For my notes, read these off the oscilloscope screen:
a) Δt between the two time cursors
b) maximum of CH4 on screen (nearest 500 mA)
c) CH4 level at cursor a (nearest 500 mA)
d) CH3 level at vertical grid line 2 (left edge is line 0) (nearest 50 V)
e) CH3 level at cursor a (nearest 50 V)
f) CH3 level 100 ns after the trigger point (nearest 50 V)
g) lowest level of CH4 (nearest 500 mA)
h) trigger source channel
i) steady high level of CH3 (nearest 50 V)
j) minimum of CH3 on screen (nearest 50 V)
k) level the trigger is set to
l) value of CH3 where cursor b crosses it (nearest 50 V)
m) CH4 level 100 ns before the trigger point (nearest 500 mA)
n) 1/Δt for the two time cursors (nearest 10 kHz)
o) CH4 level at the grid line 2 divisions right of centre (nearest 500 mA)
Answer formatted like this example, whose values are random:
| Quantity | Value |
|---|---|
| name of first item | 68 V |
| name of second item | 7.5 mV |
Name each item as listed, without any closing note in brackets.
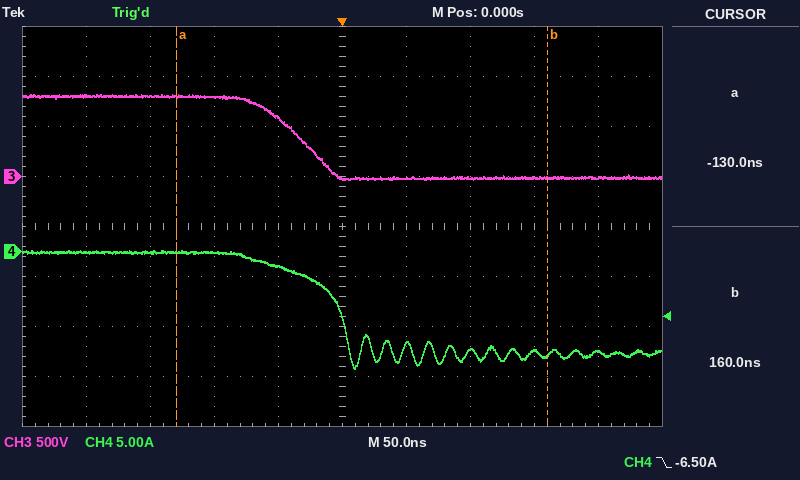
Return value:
| Quantity | Value |
|---|---|
| Δt between the two time cursors | 290 ns |
| maximum of CH4 on screen | 0.0 A |
| CH4 level at cursor a | 0.0 A |
| CH3 level at vertical grid line 2 (left edge is line 0) | 800 V |
| CH3 level at cursor a | 800 V |
| CH3 level 100 ns after the trigger point | 0 V |
| lowest level of CH4 | -11.5 A |
| trigger source channel | CH4 |
| steady high level of CH3 | 800 V |
| minimum of CH3 on screen | -50 V |
| level the trigger is set to | -6.50 A |
| value of CH3 where cursor b crosses it | 0 V |
| CH4 level 100 ns before the trigger point | 0.0 A |
| 1/Δt for the two time cursors | 3.45 MHz |
| CH4 level at the grid line 2 divisions right of centre | -10.0 A |
